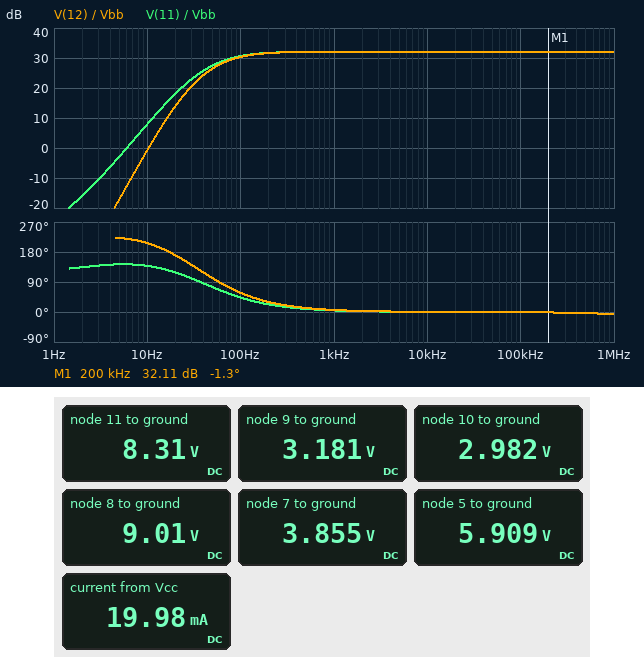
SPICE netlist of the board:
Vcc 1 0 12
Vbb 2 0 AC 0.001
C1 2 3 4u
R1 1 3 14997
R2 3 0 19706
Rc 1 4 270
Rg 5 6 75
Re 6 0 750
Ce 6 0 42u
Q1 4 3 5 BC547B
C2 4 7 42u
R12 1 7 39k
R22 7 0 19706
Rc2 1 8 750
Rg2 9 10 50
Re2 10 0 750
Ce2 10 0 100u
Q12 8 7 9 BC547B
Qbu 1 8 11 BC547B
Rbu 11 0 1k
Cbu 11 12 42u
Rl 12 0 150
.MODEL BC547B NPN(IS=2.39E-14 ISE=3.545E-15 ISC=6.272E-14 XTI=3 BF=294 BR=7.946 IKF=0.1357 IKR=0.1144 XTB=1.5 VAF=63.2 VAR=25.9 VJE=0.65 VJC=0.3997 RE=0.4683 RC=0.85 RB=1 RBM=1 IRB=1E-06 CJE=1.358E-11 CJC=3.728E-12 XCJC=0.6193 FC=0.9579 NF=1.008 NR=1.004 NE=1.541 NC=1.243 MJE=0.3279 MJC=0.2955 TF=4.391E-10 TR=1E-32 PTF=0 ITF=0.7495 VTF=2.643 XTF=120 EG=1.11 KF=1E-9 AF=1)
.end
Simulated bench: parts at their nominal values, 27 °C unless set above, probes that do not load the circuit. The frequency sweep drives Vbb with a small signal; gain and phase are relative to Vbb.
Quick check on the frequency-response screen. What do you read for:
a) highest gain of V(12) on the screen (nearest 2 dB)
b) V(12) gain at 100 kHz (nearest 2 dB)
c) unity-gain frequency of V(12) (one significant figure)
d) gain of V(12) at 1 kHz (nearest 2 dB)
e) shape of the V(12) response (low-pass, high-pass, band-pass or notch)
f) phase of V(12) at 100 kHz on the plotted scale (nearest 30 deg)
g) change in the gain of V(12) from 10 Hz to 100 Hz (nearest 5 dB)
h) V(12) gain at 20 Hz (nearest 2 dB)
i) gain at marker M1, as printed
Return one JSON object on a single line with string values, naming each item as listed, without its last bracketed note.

{"highest gain of V(12) on the screen": "32 dB", "V(12) gain at 100 kHz": "32 dB", "unity-gain frequency of V(12)": "10 Hz", "gain of V(12) at 1 kHz": "32 dB", "shape of the V(12) response": "high-pass", "phase of V(12) at 100 kHz on the plotted scale": "0 deg", "change in the gain of V(12) from 10 Hz to 100 Hz": "30 dB", "V(12) gain at 20 Hz": "14 dB", "gain at marker M1, as printed": "32.11 dB"}
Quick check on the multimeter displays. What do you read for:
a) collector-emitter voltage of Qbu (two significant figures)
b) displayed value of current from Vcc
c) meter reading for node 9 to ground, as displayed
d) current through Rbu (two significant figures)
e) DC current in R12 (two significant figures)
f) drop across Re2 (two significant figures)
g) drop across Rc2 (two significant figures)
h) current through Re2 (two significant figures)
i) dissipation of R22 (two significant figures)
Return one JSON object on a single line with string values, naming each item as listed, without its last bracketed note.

{"collector-emitter voltage of Qbu": "3.7 V", "displayed value of current from Vcc": "19.98 mA", "meter reading for node 9 to ground, as displayed": "3.181 V", "current through Rbu": "8.3 mA", "DC current in R12": "210 µA", "drop across Re2": "3.0 V", "drop across Rc2": "3.0 V", "current through Re2": "4.0 mA", "dissipation of R22": "750 µW"}
